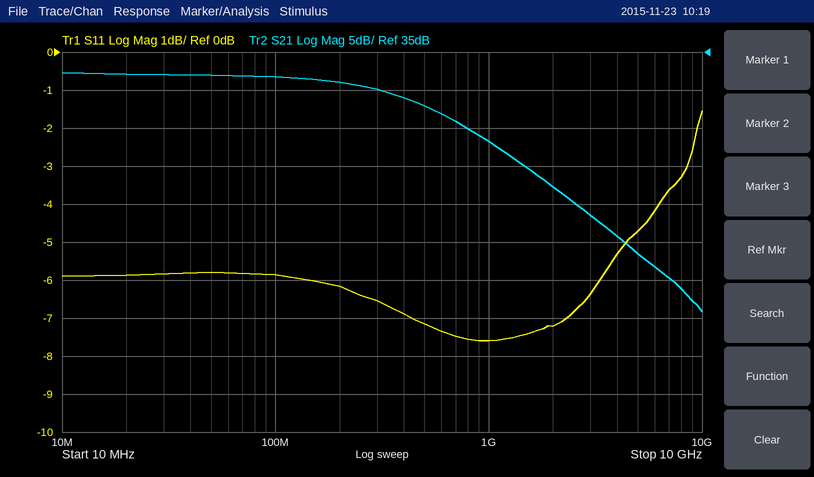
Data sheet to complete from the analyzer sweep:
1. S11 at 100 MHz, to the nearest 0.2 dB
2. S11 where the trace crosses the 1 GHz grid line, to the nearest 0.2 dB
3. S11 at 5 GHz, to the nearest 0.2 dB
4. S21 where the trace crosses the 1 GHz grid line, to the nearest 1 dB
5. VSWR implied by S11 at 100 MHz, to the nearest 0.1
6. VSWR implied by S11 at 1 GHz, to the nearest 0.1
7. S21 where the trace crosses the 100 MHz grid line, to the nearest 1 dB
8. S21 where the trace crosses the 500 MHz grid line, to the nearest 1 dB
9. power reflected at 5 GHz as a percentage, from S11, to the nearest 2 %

-5.8 dB
-7.6 dB
-4.8 dB
23 dB
3.1
2.4
32 dB
28 dB
34 %
